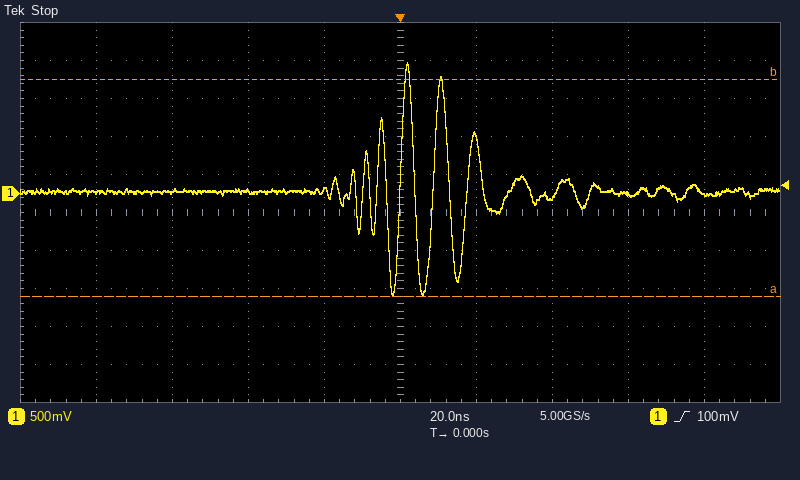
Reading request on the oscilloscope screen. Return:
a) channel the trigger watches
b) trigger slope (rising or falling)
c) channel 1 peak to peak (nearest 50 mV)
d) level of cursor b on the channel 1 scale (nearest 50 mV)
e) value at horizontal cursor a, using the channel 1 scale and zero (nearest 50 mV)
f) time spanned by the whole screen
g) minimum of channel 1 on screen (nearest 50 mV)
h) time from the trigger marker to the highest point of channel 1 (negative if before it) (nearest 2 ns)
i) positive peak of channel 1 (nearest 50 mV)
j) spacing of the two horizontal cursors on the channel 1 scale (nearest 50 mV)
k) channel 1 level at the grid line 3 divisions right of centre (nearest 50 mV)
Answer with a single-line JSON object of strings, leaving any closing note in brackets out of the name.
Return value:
{"channel the trigger watches": "channel 1", "trigger slope": "rising", "channel 1 peak to peak": "3.05 V", "level of cursor b on the channel 1 scale": "1.50 V", "value at horizontal cursor a, using the channel 1 scale and zero": "-1.35 V", "time spanned by the whole screen": "200 ns", "minimum of channel 1 on screen": "-1.35 V", "time from the trigger marker to the highest point of channel 1 (negative if before it)": "+2 ns", "positive peak of channel 1": "1.70 V", "spacing of the two horizontal cursors on the channel 1 scale": "2.85 V", "channel 1 level at the grid line 3 divisions right of centre": "0 mV"}
